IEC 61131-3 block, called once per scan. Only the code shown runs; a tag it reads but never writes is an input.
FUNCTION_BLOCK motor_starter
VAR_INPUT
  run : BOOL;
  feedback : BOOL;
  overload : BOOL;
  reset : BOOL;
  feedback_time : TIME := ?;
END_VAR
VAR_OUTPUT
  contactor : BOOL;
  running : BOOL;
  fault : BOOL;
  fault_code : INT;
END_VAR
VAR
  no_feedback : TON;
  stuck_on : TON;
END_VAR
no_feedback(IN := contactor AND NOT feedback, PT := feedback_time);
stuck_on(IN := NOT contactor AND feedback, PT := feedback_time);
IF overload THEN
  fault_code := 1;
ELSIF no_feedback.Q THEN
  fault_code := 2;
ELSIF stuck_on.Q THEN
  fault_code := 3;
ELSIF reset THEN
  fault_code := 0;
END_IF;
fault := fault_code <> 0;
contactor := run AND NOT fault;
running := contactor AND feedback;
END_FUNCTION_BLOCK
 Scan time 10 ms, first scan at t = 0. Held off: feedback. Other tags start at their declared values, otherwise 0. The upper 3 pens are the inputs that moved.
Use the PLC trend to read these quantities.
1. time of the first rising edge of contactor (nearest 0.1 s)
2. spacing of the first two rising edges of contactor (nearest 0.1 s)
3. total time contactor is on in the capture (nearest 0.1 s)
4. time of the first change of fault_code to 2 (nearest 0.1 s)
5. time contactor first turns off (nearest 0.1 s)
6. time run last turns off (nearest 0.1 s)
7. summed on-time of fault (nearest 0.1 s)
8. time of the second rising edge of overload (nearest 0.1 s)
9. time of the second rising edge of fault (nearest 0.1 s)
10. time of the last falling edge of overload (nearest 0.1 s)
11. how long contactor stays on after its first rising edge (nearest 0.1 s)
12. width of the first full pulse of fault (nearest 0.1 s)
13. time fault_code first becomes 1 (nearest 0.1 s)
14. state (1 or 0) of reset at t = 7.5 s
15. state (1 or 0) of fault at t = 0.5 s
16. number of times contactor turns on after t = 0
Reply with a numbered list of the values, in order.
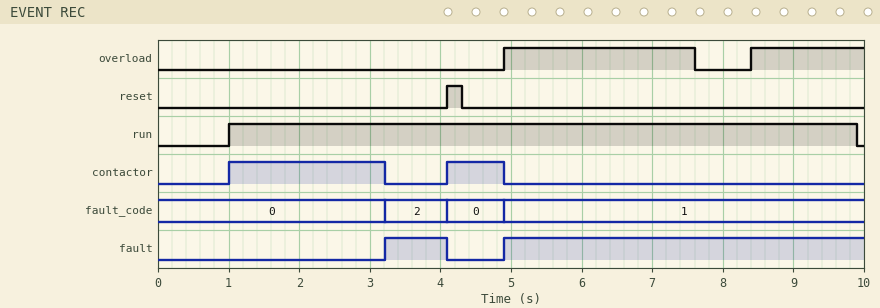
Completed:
1. 1.0 s
2. 3.1 s
3. 3.0 s
4. 3.2 s
5. 3.2 s
6. 9.9 s
7. 6.0 s
8. 8.4 s
9. 4.9 s
10. 7.6 s
11. 2.2 s
12. 0.9 s
13. 4.9 s
14. 0
15. 0
16. 2
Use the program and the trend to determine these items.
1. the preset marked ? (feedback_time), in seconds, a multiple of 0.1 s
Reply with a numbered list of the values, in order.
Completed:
1. 2.2 s
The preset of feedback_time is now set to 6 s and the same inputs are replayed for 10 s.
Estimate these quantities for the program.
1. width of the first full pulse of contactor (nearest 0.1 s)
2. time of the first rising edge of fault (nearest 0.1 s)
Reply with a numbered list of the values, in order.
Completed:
1. 3.9 s
2. 4.9 s
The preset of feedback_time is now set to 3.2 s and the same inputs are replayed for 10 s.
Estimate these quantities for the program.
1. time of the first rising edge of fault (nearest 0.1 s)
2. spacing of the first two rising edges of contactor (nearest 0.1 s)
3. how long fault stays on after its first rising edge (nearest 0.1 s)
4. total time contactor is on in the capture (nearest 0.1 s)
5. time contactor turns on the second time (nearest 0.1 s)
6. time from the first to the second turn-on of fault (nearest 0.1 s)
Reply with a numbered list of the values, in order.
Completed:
1. 4.2 s
2. 3.2 s
3. 0.0 s
4. 3.9 s
5. 4.2 s
6. 0.7 s
